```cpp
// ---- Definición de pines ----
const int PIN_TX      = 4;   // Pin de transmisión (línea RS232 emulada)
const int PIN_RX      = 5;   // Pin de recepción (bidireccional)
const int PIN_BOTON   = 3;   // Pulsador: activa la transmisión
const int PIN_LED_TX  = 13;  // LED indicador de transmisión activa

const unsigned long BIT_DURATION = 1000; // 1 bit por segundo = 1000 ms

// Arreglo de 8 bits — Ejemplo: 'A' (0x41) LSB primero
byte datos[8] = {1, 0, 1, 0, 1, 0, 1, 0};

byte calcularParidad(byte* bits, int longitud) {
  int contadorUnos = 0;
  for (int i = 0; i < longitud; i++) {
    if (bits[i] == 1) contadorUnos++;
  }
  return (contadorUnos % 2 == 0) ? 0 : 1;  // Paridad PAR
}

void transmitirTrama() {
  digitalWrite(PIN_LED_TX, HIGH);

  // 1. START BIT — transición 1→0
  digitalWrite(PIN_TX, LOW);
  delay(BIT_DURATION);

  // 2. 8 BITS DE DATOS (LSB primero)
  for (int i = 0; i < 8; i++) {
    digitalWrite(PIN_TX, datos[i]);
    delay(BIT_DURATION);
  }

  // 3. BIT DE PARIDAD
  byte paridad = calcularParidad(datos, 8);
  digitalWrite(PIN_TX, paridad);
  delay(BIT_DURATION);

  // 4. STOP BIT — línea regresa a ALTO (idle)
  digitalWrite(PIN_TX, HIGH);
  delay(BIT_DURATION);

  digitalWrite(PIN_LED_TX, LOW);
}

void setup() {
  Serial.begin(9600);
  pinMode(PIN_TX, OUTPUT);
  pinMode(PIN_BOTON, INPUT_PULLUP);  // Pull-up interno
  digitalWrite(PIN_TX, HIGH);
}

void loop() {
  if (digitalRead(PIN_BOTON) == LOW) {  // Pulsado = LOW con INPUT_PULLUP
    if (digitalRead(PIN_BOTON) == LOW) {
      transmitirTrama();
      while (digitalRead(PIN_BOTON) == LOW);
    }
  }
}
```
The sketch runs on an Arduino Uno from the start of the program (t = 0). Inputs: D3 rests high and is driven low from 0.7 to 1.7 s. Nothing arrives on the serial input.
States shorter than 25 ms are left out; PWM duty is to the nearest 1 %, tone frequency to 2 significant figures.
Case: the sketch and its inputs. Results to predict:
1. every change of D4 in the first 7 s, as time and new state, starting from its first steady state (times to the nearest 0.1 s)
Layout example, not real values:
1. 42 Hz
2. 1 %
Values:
1. 0 s high; 0.7 s low; 1.7 s high; 2.7 s low; 3.7 s high; 4.7 s low; 5.7 s high; 6.7 s low
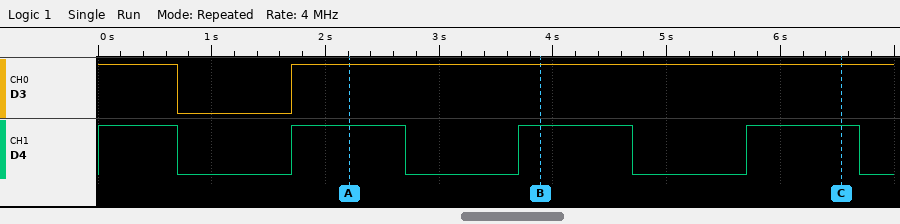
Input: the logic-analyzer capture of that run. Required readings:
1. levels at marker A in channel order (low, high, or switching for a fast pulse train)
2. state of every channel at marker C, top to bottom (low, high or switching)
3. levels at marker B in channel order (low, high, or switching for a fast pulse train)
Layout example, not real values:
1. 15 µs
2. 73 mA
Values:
1. D3 high, D4 high
2. D3 high, D4 high
3. D3 high, D4 high
